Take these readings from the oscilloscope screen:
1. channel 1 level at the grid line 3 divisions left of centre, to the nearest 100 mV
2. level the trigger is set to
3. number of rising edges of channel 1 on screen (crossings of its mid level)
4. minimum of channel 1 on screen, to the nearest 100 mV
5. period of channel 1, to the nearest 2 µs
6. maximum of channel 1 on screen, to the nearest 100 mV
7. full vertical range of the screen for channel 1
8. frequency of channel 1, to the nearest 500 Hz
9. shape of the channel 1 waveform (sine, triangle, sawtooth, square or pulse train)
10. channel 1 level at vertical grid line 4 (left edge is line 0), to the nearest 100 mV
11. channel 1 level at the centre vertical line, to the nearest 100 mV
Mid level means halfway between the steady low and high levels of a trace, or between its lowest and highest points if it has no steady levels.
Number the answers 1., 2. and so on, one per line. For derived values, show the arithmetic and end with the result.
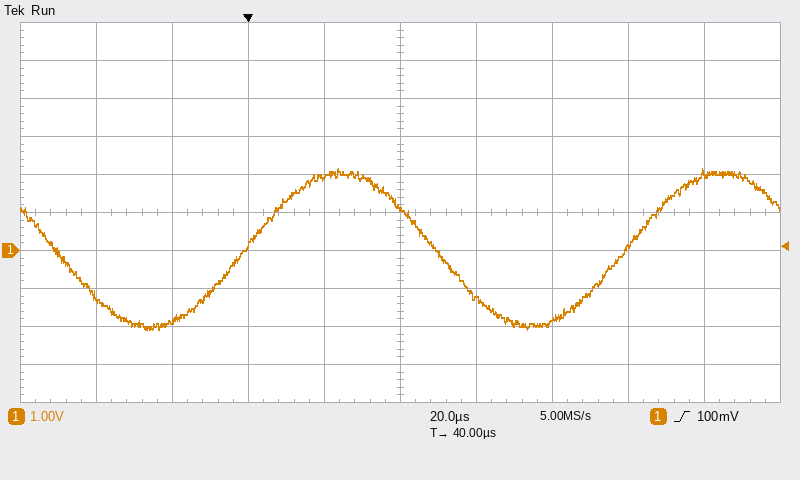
1. -1.8 V
2. 100 mV
3. 2
4. -2.1 V
5. 100 µs
6. 2.2 V
7. 10 V
8. 1 / 100 µs ≈ 10.0 kHz
9. sine
10. 1.9 V
11. 1.1 V
